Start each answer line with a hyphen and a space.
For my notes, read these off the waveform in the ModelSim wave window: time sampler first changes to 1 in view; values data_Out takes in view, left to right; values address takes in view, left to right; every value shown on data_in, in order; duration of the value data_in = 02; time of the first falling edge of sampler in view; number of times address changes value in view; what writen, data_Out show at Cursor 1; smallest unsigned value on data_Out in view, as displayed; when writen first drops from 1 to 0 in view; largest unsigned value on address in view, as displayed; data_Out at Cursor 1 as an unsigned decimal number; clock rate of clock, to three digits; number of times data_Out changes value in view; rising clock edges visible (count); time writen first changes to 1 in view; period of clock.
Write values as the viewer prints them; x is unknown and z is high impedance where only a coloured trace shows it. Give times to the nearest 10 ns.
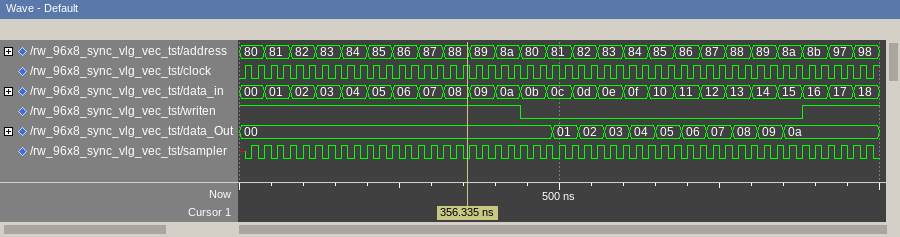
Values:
- 20 ns
- 00, 01, 02, 03, 04, 05, 06, 07, 08, 09, 0a
- 80, 81, 82, 83, 84, 85, 86, 87, 88, 89, 8a, 80, 81, 82, 83, 84, 85, 86, 87, 88, 89, 8a, 8b, 97, 98
- 00, 01, 02, 03, 04, 05, 06, 07, 08, 09, 0a, 0b, 0c, 0d, 0e, 0f, 10, 11, 12, 13, 14, 15, 16, 17, 18
- 40 ns
- 30 ns
- 24
- writen=1, data_Out=00
- 00
- 440 ns
- 98
- 0
- 50.0 MHz
- 10
- 50
- 880 ns
- 20 ns
